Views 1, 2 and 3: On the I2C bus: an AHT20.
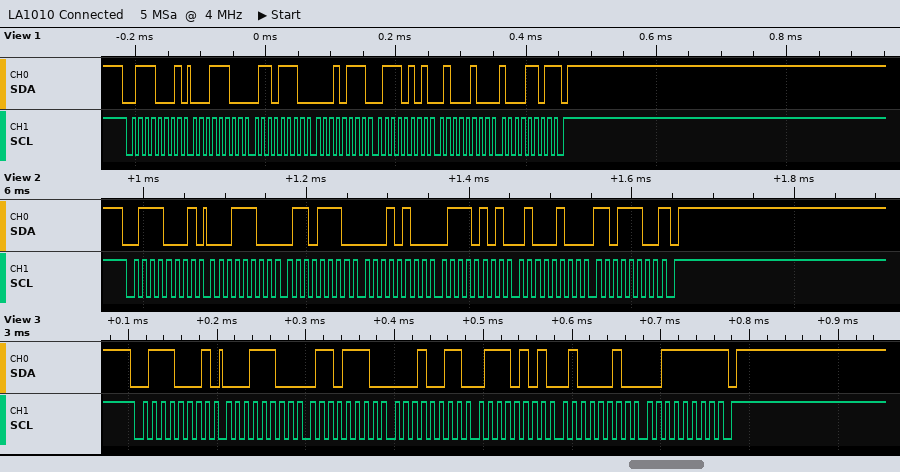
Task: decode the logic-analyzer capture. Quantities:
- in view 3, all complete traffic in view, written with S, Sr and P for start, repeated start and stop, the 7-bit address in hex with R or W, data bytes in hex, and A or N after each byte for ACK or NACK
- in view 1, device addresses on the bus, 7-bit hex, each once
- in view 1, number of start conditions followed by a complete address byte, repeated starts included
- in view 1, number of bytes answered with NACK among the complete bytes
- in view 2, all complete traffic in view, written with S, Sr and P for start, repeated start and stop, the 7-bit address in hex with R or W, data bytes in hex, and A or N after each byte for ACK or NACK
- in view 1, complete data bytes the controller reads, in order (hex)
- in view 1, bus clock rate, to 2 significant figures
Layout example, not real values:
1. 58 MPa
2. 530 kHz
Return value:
1. S 38R A 1C A 6E A 13 A 75 A 42 A 3F N P
2. 0x38
3. 1
4. 1
5. S 38R A 1C A 6E A 14 A 75 A 44 A DC N P
6. 1C 6E 17 75 44 8D
7. 100 kHz
